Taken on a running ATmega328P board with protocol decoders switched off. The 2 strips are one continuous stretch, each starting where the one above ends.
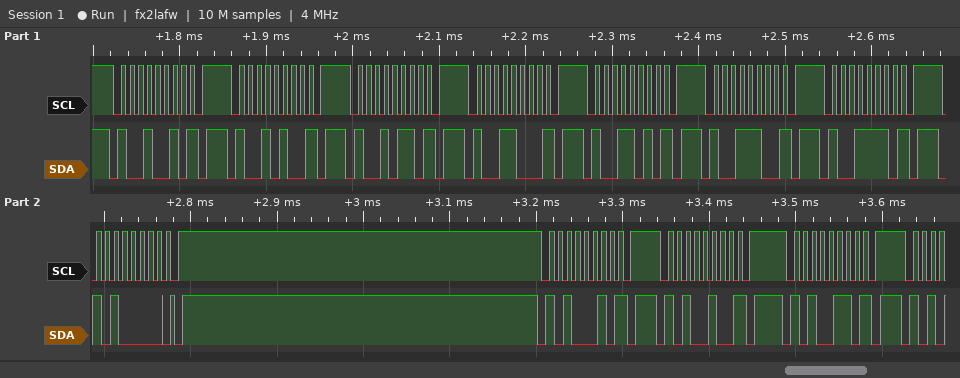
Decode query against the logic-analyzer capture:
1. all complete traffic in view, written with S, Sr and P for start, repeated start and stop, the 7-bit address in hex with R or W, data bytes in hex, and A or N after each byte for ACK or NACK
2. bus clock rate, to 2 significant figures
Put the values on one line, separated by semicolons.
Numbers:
S 49W N P S 4AW N P S 4BW N P S 4CW N P S 4DW N P S 4EW N P S 4FW N P S 50W A P S 51W N P S 52W N P S 53W N P; 100 kHz
